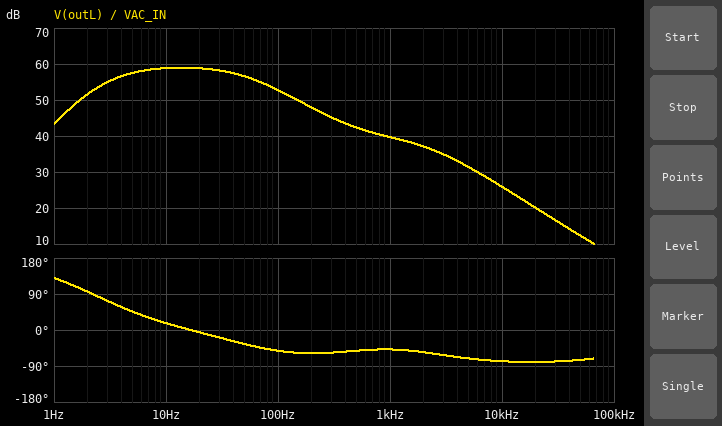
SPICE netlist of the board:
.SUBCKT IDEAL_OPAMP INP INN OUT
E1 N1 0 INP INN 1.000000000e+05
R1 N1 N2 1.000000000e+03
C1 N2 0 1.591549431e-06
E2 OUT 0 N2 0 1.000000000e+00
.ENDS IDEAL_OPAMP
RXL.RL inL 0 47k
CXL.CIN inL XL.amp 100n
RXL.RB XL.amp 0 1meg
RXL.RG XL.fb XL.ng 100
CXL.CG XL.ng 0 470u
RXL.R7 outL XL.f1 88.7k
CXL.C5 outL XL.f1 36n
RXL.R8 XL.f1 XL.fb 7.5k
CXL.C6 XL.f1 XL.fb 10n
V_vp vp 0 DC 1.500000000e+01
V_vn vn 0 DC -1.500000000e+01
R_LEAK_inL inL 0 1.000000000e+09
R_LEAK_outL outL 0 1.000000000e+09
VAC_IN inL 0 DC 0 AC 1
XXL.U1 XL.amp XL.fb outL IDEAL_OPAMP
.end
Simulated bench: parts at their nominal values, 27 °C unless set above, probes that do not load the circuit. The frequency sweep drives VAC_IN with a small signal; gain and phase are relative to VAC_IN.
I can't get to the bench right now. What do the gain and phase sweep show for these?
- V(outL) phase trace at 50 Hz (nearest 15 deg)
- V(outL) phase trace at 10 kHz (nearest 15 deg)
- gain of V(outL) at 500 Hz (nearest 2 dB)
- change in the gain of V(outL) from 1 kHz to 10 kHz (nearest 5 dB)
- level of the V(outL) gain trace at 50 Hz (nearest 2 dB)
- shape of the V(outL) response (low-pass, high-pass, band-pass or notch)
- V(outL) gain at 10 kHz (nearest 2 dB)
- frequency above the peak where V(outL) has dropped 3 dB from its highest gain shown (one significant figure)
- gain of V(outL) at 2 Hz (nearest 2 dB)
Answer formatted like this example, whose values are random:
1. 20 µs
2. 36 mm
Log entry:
1. -30 deg
2. -75 deg
3. 42 dB
4. -15 dB
5. 56 dB
6. band-pass
7. 26 dB
8. 60 Hz
9. 52 dB
